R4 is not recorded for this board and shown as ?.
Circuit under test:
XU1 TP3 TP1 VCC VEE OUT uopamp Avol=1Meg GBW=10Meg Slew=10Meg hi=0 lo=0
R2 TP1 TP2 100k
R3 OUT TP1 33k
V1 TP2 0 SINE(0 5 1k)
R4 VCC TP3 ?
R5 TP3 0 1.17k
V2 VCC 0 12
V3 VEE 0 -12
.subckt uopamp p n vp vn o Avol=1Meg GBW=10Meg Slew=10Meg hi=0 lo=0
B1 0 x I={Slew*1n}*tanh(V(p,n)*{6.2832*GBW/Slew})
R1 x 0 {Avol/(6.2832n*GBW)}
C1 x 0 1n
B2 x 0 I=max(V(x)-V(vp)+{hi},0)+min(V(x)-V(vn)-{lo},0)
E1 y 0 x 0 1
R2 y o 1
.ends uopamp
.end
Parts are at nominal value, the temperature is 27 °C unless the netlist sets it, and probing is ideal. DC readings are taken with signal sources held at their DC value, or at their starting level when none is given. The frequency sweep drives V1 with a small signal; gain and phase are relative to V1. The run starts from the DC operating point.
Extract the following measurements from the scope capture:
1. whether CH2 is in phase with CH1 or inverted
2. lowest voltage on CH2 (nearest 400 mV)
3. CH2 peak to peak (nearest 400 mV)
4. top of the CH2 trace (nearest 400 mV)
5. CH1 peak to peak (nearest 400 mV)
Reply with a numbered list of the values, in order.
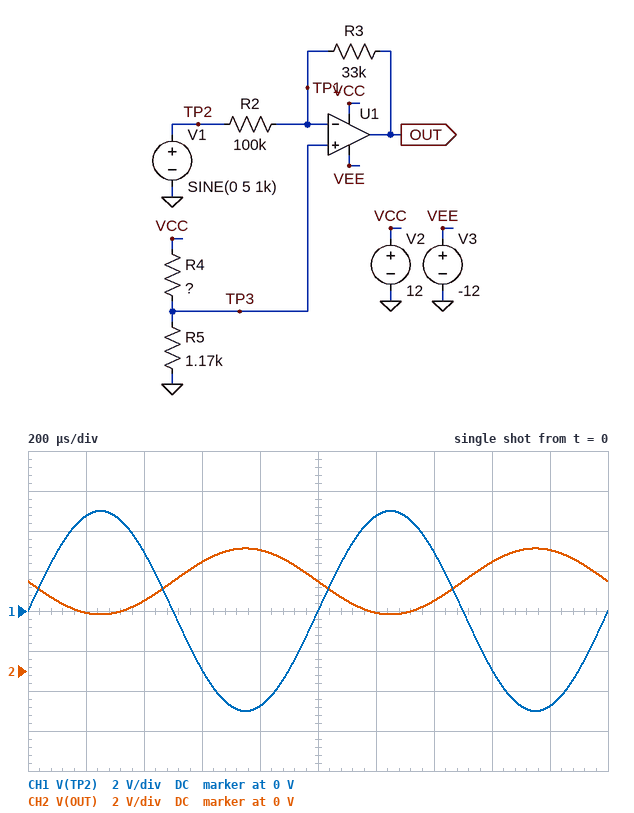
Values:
1. inverted
2. 2.8 V
3. 3.2 V
4. 6.0 V
5. 10.0 V
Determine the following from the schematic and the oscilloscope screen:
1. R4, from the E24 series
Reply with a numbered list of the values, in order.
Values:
1. 3 kΩ
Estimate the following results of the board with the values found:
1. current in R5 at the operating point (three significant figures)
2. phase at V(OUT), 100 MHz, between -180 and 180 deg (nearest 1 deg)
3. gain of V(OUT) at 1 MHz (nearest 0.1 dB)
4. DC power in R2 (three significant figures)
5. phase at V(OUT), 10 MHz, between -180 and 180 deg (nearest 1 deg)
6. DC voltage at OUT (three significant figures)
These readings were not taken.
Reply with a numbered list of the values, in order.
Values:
1. 2.88 mA
2. 94 deg
3. -9.7 dB
4. 113 µW
5. 127 deg
6. 4.48 V
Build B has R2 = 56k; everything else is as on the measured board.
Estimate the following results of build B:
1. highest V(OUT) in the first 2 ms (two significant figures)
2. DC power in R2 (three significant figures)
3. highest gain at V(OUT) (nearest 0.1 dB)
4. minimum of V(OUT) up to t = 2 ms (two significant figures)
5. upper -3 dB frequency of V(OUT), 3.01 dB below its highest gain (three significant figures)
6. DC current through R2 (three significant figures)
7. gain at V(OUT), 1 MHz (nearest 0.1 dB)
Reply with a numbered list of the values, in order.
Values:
1. 8.3 V
2. 202 µW
3. -4.6 dB
4. 2.4 V
5. 6.29 MHz
6. 60.1 µA
7. -4.7 dB
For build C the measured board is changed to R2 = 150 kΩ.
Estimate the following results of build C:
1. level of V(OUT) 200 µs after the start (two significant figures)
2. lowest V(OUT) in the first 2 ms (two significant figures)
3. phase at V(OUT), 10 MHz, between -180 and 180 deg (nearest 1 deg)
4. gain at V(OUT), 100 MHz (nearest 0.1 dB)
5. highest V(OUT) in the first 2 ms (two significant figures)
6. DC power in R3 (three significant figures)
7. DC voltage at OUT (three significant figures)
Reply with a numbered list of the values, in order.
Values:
1. 3.1 V
2. 3.0 V
3. 129 deg
4. -34.9 dB
5. 5.2 V
6. 16.6 µW
7. 4.11 V
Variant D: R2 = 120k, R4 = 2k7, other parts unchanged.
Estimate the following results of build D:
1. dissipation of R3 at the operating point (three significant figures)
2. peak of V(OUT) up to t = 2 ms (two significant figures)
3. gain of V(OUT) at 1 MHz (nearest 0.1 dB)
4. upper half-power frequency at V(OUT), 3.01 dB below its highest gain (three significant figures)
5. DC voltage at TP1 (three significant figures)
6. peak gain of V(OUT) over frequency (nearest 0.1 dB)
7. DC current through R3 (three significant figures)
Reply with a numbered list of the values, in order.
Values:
1. 30.2 µW
2. 6.0 V
3. -11.3 dB
4. 7.84 MHz
5. 3.63 V
6. -11.2 dB
7. 30.2 µA
